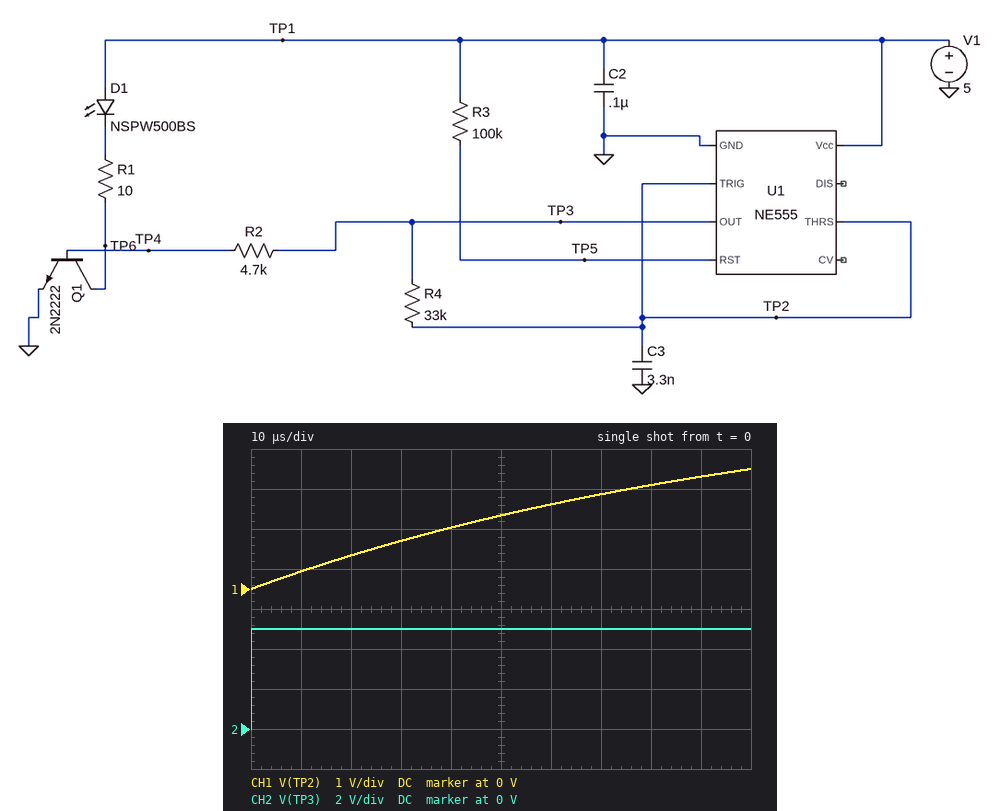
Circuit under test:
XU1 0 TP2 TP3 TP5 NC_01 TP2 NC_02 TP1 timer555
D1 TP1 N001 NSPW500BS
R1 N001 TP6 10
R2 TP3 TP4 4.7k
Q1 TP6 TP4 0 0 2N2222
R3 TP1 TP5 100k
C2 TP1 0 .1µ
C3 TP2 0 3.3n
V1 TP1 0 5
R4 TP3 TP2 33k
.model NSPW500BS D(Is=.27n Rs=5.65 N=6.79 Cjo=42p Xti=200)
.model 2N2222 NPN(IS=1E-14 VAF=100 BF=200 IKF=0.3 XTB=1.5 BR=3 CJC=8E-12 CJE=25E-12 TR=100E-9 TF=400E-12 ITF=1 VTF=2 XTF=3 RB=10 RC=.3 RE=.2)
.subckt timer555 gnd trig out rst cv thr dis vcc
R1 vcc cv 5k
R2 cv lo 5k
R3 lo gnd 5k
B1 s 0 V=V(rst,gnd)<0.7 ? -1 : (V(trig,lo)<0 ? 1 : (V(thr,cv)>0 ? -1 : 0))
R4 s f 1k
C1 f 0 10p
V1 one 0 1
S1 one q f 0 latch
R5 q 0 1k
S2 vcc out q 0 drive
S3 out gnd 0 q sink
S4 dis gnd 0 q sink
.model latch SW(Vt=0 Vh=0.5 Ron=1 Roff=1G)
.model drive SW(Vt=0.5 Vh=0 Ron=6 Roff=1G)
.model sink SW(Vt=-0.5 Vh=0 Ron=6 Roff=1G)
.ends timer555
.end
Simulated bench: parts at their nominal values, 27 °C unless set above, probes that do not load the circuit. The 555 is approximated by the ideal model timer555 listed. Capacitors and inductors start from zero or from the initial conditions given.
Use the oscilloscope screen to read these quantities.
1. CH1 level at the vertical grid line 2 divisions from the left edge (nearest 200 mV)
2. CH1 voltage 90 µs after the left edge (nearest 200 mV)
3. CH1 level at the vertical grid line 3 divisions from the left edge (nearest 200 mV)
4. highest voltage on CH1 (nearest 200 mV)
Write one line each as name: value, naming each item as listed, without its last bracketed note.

CH1 level at the vertical grid line 2 divisions from the left edge: 800 mV
CH1 voltage 90 µs after the left edge: 2.8 V
CH1 level at the vertical grid line 3 divisions from the left edge: 1.2 V
highest voltage on CH1: 3.0 V
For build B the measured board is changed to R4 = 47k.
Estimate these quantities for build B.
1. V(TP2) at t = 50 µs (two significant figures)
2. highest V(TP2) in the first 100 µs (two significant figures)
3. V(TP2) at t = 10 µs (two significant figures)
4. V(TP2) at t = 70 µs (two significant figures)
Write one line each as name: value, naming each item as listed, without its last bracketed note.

V(TP2) at t = 50 µs: 1.4 V
highest V(TP2) in the first 100 µs: 2.4 V
V(TP2) at t = 10 µs: 310 mV
V(TP2) at t = 70 µs: 1.8 V
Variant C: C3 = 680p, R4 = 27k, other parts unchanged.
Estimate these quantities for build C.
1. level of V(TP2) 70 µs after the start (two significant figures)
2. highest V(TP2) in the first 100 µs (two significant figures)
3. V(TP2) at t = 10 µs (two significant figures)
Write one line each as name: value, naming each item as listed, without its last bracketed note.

level of V(TP2) 70 µs after the start: 3.2 V
highest V(TP2) in the first 100 µs: 3.3 V
V(TP2) at t = 10 µs: 2.1 V
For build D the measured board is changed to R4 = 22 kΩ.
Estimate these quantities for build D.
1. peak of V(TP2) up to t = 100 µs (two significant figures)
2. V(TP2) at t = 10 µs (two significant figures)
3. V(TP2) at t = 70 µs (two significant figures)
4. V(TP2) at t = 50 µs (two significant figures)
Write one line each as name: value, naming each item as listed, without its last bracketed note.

peak of V(TP2) up to t = 100 µs: 3.3 V
V(TP2) at t = 10 µs: 640 mV
V(TP2) at t = 70 µs: 3.1 V
V(TP2) at t = 50 µs: 2.5 V
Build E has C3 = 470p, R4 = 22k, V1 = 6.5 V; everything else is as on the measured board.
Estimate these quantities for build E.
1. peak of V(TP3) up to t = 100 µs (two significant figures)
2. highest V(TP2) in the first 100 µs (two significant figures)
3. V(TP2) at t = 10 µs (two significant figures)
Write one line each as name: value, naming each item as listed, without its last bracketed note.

peak of V(TP3) up to t = 100 µs: 6.5 V
highest V(TP2) in the first 100 µs: 4.3 V
V(TP2) at t = 10 µs: 4.0 V
